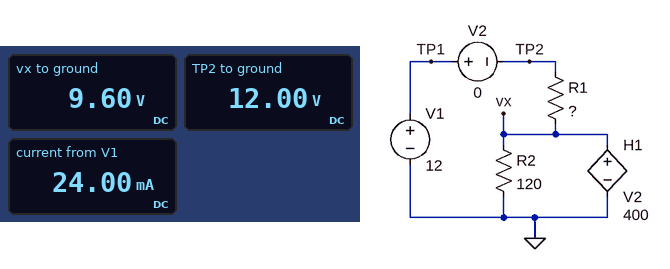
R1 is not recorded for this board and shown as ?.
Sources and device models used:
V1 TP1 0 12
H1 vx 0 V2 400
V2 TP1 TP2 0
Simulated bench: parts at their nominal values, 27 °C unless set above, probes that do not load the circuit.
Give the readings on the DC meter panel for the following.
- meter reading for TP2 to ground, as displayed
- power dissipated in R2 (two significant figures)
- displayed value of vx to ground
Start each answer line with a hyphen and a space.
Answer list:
- 12.00 V
- 770 mW
- 9.60 V
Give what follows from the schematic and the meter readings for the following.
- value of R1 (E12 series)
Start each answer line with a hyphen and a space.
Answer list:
- 100 Ω
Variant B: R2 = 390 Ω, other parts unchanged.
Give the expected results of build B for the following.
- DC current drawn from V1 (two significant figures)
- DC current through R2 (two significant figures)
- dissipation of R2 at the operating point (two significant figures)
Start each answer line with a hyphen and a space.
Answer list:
- 24 mA
- 25 mA
- 240 mW
